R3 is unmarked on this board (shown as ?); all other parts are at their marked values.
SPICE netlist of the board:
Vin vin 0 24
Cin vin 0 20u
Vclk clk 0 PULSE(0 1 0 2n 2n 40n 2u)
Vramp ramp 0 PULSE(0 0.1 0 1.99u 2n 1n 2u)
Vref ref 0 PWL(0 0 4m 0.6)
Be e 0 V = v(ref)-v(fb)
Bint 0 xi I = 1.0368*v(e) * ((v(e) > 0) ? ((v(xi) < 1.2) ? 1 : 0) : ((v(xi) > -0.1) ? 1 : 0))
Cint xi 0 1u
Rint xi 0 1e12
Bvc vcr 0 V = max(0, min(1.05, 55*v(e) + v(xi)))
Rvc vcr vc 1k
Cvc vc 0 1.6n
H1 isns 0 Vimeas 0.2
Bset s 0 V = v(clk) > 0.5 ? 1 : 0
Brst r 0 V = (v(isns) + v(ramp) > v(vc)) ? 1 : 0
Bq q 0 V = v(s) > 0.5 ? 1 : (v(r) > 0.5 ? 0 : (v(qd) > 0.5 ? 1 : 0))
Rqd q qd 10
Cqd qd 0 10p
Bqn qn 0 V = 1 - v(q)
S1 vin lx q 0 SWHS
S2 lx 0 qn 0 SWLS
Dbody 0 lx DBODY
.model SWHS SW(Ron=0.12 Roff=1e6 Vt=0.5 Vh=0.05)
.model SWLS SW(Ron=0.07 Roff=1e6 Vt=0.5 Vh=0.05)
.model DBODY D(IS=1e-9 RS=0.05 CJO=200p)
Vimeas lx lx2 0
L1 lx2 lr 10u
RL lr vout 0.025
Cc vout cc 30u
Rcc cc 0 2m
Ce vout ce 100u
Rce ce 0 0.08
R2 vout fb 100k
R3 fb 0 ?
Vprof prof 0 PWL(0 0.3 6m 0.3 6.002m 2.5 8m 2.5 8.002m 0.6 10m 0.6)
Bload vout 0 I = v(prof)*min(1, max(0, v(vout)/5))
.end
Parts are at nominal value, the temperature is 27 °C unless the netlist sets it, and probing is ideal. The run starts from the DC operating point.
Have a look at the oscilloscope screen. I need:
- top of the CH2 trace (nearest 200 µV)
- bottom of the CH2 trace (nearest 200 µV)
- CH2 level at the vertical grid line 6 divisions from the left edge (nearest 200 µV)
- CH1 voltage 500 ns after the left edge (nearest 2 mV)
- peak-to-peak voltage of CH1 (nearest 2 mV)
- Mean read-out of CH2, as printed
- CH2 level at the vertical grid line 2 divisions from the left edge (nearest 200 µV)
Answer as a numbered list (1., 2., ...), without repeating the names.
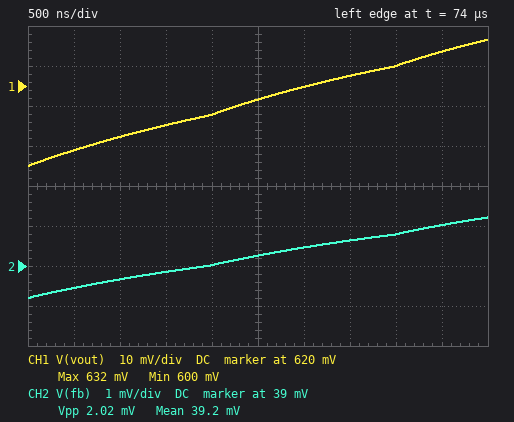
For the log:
1. 40.2 mV
2. 38.2 mV
3. 39.4 mV
4. 604 mV
5. 32 mV
6. 39.2 mV
7. 38.6 mV
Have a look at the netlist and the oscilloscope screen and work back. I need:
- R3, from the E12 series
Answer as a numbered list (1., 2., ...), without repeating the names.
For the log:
1. 6.8 kΩ
